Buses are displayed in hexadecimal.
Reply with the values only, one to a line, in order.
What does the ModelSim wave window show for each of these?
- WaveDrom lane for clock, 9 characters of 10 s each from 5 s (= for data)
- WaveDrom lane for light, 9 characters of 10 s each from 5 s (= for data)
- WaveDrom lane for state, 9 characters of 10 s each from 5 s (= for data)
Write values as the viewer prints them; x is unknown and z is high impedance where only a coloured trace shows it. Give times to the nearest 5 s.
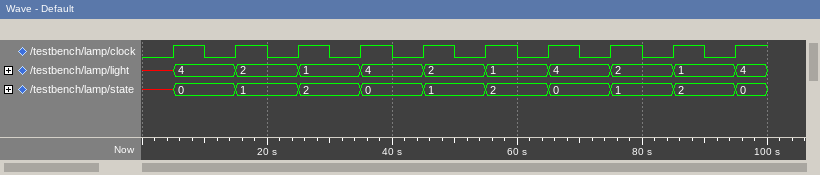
{name: 'clock', wave: 'p........'}
{name: 'light', wave: '=========', data: '4 2 1 4 2 1 4 2 1'}
{name: 'state', wave: '=========', data: '0 1 2 0 1 2 0 1 2'}
